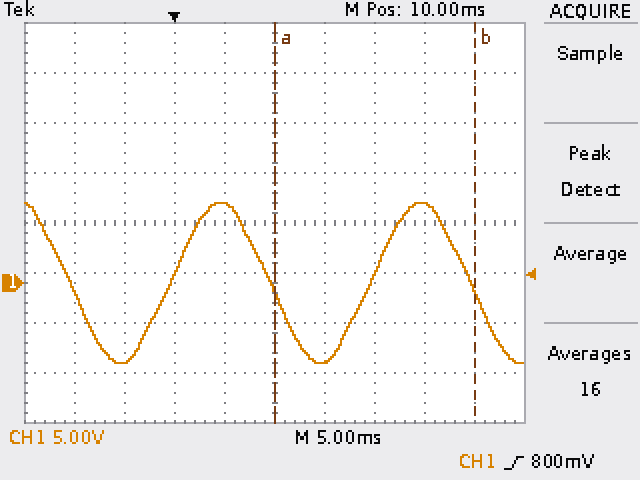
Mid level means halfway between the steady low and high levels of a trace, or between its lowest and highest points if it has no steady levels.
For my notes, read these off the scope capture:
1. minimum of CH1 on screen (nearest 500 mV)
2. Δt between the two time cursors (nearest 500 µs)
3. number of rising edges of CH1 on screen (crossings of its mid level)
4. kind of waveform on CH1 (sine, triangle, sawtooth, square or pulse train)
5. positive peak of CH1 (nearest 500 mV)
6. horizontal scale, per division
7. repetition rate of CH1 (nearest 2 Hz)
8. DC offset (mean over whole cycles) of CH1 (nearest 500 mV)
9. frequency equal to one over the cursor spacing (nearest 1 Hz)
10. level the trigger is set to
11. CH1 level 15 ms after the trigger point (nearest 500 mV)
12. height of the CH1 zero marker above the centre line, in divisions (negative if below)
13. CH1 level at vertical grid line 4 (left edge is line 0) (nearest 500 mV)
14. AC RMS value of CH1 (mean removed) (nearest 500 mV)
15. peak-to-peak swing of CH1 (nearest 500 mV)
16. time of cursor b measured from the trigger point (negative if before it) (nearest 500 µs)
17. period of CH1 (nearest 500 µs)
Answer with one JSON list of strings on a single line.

["-8.0 V", "20.0 ms", "2", "sine", "8.0 V", "5 ms", "50 Hz", "0.0 V", "50 Hz", "800 mV", "-8.0 V", "-1.2 div", "8.0 V", "5.5 V", "16.0 V", "+30.0 ms", "20.0 ms"]
